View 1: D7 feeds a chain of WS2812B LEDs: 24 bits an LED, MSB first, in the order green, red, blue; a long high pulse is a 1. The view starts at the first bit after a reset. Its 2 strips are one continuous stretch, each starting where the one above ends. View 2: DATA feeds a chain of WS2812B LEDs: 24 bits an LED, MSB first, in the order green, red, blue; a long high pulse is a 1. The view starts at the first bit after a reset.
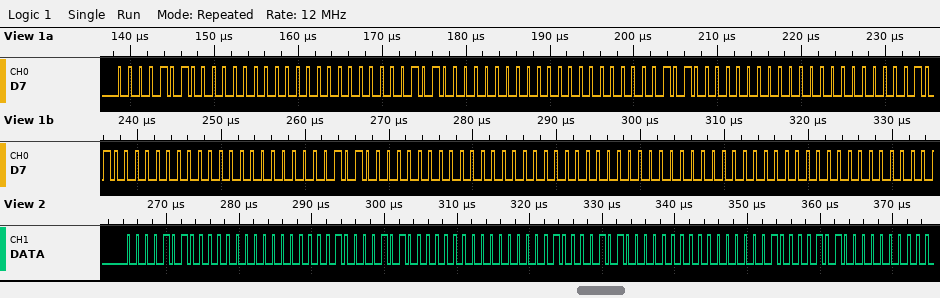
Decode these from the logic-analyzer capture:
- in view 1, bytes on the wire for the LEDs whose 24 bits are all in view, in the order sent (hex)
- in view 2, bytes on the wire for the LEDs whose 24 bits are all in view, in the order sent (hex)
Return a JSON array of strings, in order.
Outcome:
["0A 00 00 0A 00 00 0A 00 00 0A 00 00 0A 00 00 00 00 00", "0A 00 01 0A 00 01 0A 00 01"]
